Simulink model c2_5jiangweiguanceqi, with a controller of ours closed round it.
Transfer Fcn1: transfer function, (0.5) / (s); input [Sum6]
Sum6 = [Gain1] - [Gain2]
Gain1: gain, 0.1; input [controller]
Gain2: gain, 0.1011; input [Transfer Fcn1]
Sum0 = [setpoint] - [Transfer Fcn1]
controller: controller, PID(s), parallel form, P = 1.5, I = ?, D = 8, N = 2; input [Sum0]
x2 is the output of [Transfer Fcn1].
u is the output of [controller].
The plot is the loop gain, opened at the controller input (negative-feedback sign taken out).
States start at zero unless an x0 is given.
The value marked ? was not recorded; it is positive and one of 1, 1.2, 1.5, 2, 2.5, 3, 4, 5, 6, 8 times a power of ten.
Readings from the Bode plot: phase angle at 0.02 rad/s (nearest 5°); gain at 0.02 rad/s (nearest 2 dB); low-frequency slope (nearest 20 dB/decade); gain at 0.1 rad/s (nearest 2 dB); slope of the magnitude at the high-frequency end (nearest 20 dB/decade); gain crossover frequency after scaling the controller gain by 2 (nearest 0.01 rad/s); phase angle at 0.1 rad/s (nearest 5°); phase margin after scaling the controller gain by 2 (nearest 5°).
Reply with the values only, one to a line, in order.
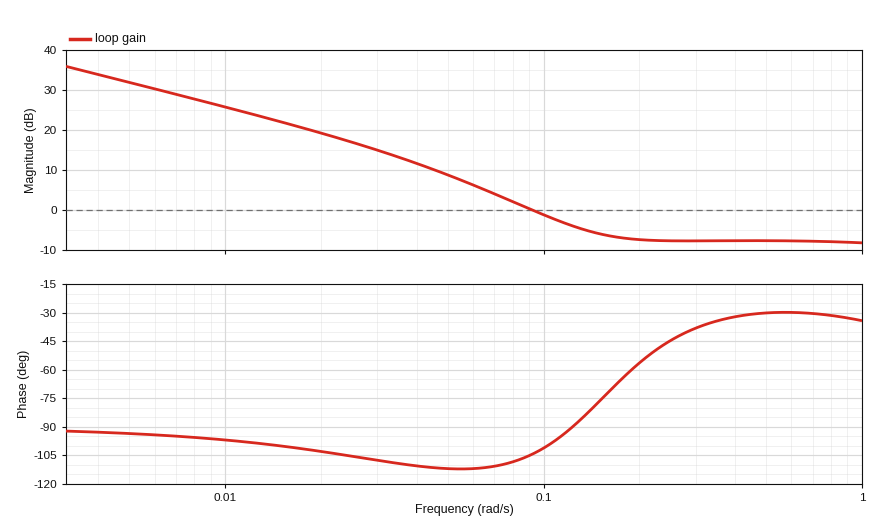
-105°
20 dB
-20 dB/decade
-2 dB
0 dB/decade
0.15 rad/s
-100°
105°
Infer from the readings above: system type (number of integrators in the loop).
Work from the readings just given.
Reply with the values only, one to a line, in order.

1
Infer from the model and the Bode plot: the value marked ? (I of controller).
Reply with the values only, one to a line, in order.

0.2
